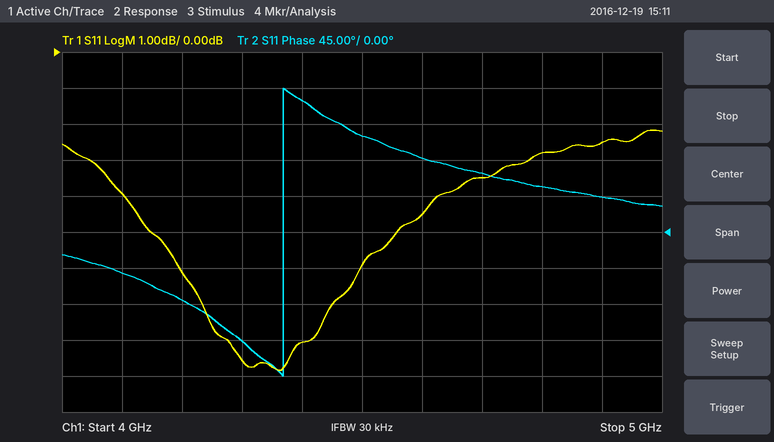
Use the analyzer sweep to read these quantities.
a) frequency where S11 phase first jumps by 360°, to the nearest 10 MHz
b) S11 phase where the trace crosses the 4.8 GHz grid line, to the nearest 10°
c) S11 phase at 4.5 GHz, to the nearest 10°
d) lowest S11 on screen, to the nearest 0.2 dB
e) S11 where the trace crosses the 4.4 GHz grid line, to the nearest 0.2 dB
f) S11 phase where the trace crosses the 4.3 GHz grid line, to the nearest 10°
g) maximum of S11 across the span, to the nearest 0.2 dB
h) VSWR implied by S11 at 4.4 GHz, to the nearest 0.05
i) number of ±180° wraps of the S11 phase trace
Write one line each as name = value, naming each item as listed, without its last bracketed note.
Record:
frequency where S11 phase first jumps by 360°, to the nearest 10 MHz = 4.37 GHz
S11 phase where the trace crosses the 4.8 GHz grid line, to the nearest 10° = 60°
S11 phase at 4.5 GHz, to the nearest 10° = 120°
lowest S11 on screen, to the nearest 0.2 dB = -8.8 dB
S11 where the trace crosses the 4.4 GHz grid line, to the nearest 0.2 dB = -8.0 dB
S11 phase where the trace crosses the 4.3 GHz grid line, to the nearest 10° = -140°
maximum of S11 across the span, to the nearest 0.2 dB = -2.2 dB
VSWR implied by S11 at 4.4 GHz, to the nearest 0.05 = 2.30
number of ±180° wraps of the S11 phase trace = 1
